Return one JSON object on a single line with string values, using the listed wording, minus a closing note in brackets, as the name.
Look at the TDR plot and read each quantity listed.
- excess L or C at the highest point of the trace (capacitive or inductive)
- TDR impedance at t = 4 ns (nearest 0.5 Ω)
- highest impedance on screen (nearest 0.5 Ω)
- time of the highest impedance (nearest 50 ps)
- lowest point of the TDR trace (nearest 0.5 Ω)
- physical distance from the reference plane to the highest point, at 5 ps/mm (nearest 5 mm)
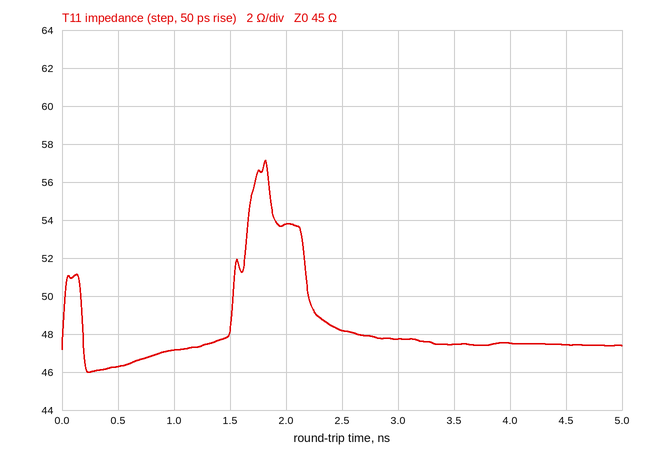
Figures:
{"excess L or C at the highest point of the trace": "inductive", "TDR impedance at t = 4 ns": "47.5 Ω", "highest impedance on screen": "57.0 Ω", "time of the highest impedance": "1.80 ns", "lowest point of the TDR trace": "46.0 Ω", "physical distance from the reference plane to the highest point, at 5 ps/mm": "180 mm"}
